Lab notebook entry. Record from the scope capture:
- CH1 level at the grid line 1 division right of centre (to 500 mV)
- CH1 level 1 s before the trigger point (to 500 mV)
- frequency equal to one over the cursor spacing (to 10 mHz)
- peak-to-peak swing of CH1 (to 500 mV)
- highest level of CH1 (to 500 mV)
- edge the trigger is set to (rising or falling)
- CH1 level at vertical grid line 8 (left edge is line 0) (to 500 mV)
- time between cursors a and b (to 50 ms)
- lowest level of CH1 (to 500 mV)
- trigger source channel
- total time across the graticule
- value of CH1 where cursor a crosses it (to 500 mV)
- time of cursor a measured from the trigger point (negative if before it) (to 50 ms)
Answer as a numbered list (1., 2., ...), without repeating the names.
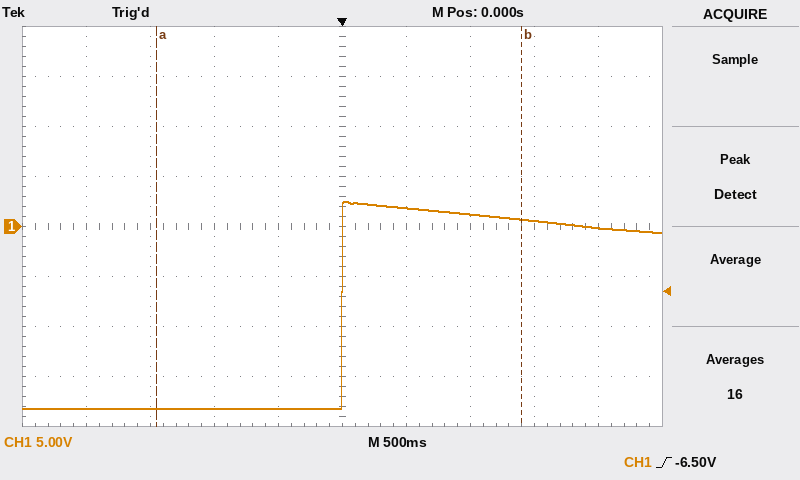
1. 2.0 V
2. -18.0 V
3. 350 mHz
4. 20.5 V
5. 2.5 V
6. rising
7. 500 mV
8. 2.85 s
9. -18.0 V
10. CH1
11. 5 s
12. -18.0 V
13. -1.45 s
